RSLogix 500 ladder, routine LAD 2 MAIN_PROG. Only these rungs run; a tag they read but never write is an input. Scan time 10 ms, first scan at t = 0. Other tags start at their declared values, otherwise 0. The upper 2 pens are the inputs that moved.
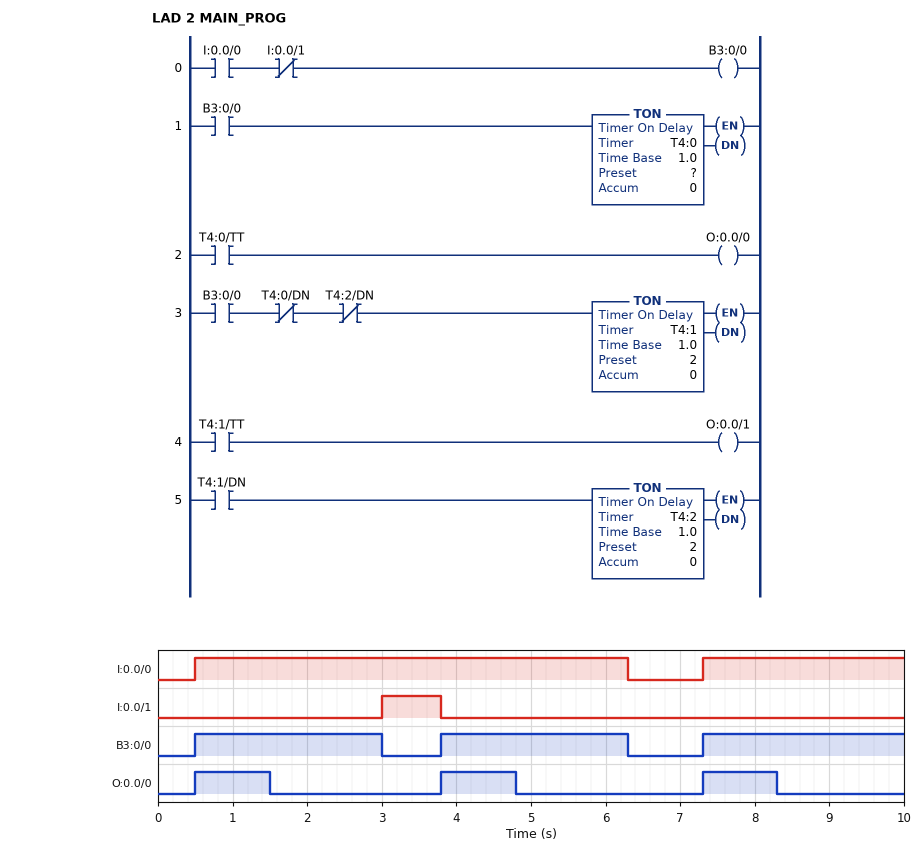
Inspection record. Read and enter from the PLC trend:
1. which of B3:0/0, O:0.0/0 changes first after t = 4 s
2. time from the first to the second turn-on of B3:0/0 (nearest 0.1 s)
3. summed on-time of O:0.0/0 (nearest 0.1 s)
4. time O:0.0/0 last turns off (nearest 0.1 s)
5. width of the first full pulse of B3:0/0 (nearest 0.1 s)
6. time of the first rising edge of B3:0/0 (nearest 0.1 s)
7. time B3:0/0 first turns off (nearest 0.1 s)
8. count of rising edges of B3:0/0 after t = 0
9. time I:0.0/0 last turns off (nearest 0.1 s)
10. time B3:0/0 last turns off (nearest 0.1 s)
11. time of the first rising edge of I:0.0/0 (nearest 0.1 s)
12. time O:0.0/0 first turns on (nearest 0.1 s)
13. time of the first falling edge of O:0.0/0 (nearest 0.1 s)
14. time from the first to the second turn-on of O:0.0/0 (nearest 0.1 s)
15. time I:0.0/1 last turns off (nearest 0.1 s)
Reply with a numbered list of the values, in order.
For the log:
1. O:0.0/0
2. 3.3 s
3. 3.0 s
4. 8.3 s
5. 2.5 s
6. 0.5 s
7. 3.0 s
8. 3
9. 6.3 s
10. 6.3 s
11. 0.5 s
12. 0.5 s
13. 1.5 s
14. 3.3 s
15. 3.8 s
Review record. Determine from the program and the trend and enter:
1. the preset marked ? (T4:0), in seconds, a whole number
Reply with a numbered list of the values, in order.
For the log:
1. 1 s
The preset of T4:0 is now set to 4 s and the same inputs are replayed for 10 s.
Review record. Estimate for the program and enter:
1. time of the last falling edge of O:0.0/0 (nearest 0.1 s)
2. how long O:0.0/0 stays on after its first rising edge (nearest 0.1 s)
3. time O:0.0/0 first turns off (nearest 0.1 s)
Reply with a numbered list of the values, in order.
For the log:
1. 6.3 s
2. 2.5 s
3. 3.0 s
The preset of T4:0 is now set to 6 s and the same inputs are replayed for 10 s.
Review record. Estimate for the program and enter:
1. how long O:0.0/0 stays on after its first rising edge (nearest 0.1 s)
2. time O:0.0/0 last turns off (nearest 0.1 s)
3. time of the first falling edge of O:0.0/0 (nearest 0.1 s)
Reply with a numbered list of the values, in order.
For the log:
1. 2.5 s
2. 6.3 s
3. 3.0 s
